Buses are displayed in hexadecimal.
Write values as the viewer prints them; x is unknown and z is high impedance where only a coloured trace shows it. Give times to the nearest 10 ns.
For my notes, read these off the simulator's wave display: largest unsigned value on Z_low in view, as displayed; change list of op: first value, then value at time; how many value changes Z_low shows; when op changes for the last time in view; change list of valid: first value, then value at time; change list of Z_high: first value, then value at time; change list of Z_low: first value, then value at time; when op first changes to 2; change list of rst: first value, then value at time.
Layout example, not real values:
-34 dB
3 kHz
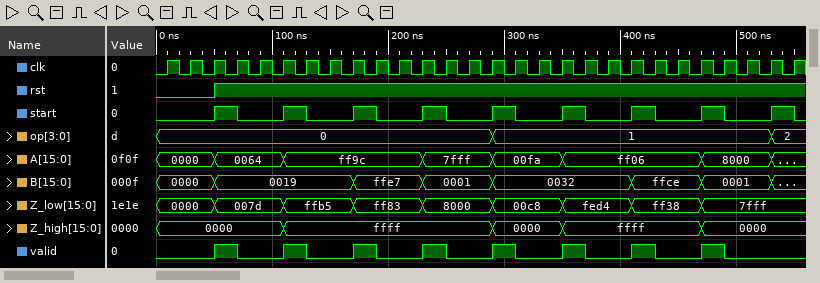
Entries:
ffb5
0, 1 at 290 ns, 2 at 530 ns
8
530 ns
0, 1 at 50 ns, 0 at 70 ns, 1 at 110 ns, 0 at 130 ns, 1 at 170 ns, 0 at 190 ns, 1 at 230 ns, 0 at 250 ns, 1 at 290 ns, 0 at 310 ns, 1 at 350 ns, 0 at 370 ns, 1 at 410 ns, 0 at 430 ns, 1 at 470 ns, 0 at 490 ns
0000, ffff at 110 ns, 0000 at 290 ns, ffff at 350 ns, 0000 at 470 ns
0000, 007d at 50 ns, ffb5 at 110 ns, ff83 at 170 ns, 8000 at 230 ns, 00c8 at 290 ns, fed4 at 350 ns, ff38 at 410 ns, 7fff at 470 ns
530 ns
0, 1 at 50 ns
